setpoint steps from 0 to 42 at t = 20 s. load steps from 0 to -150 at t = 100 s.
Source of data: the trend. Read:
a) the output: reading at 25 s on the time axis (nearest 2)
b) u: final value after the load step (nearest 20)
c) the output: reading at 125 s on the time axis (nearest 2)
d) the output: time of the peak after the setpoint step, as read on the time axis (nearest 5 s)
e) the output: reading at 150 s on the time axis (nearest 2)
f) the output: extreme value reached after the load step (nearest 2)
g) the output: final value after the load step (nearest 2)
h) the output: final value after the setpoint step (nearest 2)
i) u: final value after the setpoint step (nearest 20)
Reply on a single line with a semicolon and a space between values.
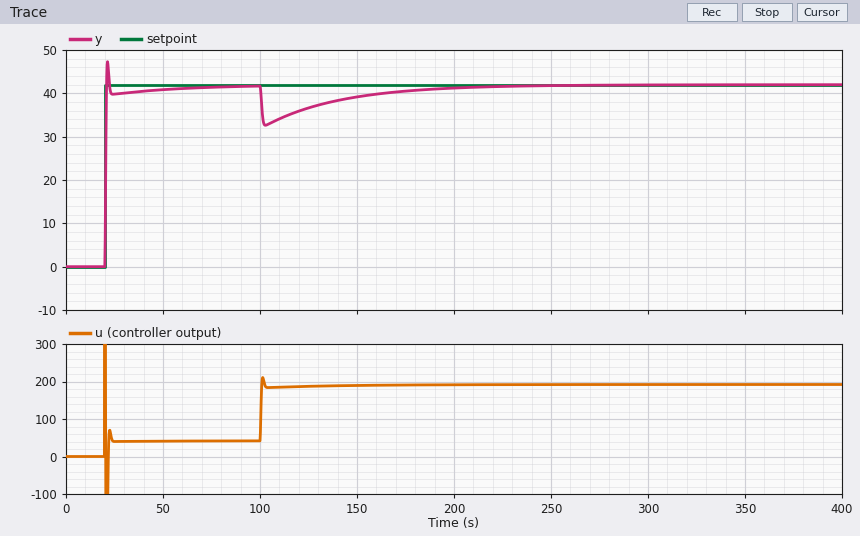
40; 200; 36; 20 s; 40; 32; 42; 42; 40
